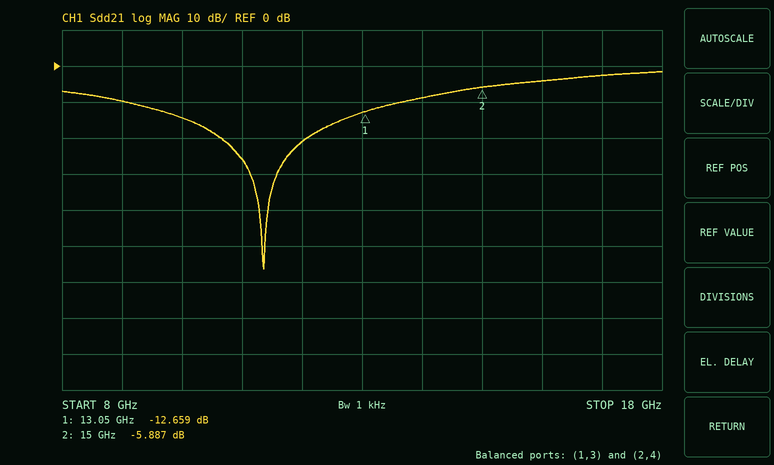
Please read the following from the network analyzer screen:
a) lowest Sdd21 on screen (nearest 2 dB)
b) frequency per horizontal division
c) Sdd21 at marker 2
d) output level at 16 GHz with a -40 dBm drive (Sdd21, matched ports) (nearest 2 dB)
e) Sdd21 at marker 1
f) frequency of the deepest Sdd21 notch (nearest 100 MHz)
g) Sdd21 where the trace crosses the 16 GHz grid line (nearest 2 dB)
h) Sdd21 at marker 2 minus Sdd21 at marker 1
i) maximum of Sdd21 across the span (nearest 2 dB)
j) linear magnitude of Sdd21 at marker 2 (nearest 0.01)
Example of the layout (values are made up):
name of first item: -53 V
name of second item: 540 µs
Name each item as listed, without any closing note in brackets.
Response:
lowest Sdd21 on screen: -56 dB
frequency per horizontal division: 1 GHz
Sdd21 at marker 2: -5.887 dB
output level at 16 GHz with a -40 dBm drive (Sdd21, matched ports): -44 dBm
Sdd21 at marker 1: -12.659 dB
frequency of the deepest Sdd21 notch: 11.4 GHz
Sdd21 where the trace crosses the 16 GHz grid line: -4 dB
Sdd21 at marker 2 minus Sdd21 at marker 1: 6.772 dB
maximum of Sdd21 across the span: -2 dB
linear magnitude of Sdd21 at marker 2: 0.51
